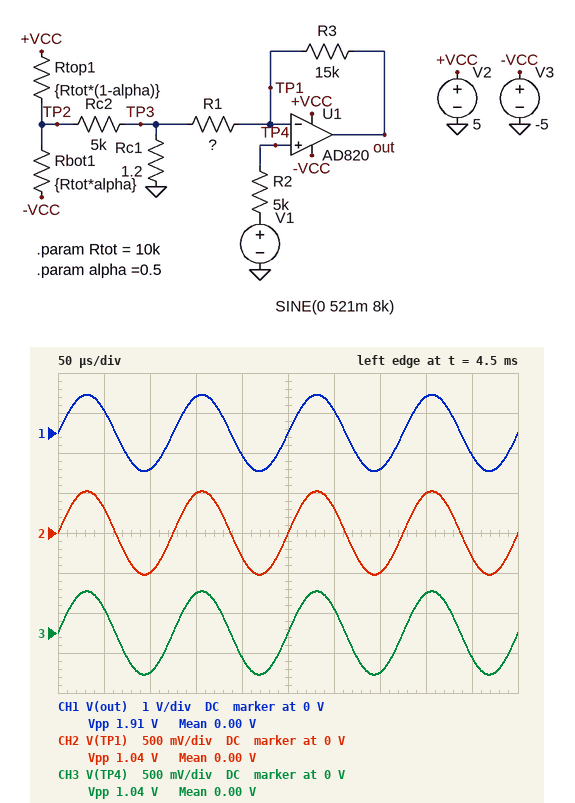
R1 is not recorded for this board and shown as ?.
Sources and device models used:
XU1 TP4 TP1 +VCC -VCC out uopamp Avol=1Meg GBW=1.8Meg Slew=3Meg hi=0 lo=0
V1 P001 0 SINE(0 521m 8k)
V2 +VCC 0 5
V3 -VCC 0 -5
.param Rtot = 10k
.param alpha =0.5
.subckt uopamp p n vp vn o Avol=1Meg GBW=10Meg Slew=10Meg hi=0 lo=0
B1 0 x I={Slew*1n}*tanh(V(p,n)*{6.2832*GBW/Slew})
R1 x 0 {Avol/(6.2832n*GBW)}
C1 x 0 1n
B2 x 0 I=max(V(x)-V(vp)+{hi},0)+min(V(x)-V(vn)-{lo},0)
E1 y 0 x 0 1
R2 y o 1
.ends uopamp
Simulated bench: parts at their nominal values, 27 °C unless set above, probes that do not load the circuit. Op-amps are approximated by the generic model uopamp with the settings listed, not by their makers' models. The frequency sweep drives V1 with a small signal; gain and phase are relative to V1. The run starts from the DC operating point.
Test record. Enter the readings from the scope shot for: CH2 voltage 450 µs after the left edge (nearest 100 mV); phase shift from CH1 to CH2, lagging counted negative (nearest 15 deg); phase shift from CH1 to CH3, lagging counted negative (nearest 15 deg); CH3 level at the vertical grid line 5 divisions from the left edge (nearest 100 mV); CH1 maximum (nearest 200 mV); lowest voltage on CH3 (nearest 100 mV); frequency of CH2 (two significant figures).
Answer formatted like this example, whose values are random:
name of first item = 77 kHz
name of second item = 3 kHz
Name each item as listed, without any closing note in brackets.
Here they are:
CH2 voltage 450 µs after the left edge = -300 mV
phase shift from CH1 to CH2, lagging counted negative = 0 deg
phase shift from CH1 to CH3, lagging counted negative = 0 deg
CH3 level at the vertical grid line 5 divisions from the left edge = 0 V
CH1 maximum = 1.0 V
lowest voltage on CH3 = -500 mV
frequency of CH2 = 8.0 kHz
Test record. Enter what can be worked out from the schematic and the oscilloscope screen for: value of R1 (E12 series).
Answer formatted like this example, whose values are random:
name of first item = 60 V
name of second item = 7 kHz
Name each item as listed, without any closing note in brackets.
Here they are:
value of R1 = 18 kΩ
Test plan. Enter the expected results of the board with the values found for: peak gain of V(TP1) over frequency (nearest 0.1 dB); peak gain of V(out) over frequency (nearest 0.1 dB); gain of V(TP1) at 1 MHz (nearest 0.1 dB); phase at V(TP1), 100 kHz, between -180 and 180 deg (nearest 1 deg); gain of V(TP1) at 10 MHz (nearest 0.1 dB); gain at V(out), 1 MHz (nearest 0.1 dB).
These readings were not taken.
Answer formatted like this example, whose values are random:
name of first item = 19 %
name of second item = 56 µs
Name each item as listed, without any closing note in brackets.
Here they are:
peak gain of V(TP1) over frequency = 0 dB
peak gain of V(out) over frequency = 5.3 dB
gain of V(TP1) at 1 MHz = -3.1 dB
phase at V(TP1), 100 kHz, between -180 and 180 deg = -6 deg
gain of V(TP1) at 10 MHz = -20.2 dB
gain at V(out), 1 MHz = 2.2 dB
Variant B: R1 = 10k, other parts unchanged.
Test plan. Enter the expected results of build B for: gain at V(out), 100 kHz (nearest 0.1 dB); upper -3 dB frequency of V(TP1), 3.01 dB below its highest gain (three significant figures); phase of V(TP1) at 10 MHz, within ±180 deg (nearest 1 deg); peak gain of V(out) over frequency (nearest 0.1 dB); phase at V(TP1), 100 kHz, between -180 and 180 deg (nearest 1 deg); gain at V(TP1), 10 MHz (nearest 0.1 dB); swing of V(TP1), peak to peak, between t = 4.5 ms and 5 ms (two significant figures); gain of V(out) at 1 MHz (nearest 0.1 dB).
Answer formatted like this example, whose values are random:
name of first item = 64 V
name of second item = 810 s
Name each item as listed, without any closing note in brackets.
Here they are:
gain at V(out), 100 kHz = 7.9 dB
upper -3 dB frequency of V(TP1), 3.01 dB below its highest gain = 720 kHz
phase of V(TP1) at 10 MHz, within ±180 deg = -86 deg
peak gain of V(out) over frequency = 8.0 dB
phase at V(TP1), 100 kHz, between -180 and 180 deg = -8 deg
gain at V(TP1), 10 MHz = -22.9 dB
swing of V(TP1), peak to peak, between t = 4.5 ms and 5 ms = 1.0 V
gain of V(out) at 1 MHz = 3.3 dB
